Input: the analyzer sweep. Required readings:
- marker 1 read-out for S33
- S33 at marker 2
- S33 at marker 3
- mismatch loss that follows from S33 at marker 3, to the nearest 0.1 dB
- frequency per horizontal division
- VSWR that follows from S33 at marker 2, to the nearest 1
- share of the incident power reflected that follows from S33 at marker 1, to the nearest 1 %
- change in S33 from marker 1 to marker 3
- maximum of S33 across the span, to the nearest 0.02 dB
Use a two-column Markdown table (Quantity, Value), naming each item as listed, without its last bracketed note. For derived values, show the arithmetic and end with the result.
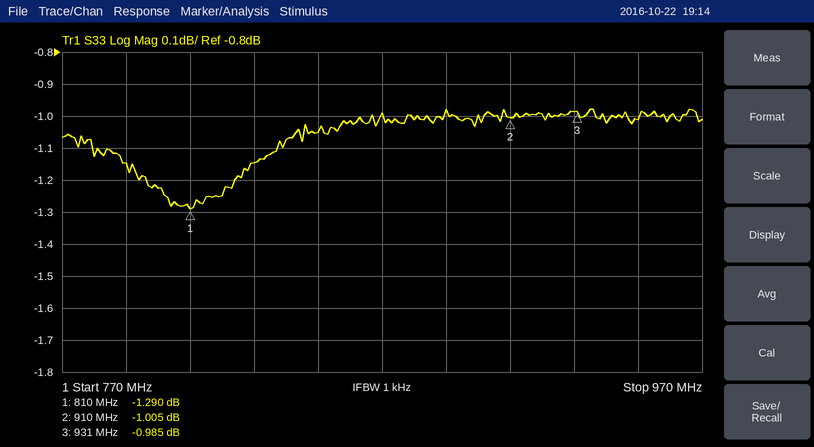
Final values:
| Quantity | Value |
|---|---|
| marker 1 read-out for S33 | -1.290 dB |
| S33 at marker 2 | -1.005 dB |
| S33 at marker 3 | -0.985 dB |
| mismatch loss that follows from S33 at marker 3, to the nearest 0.1 dB | −10 log10(1 − 10^(-0.985/10)) ≈ 6.9 dB |
| frequency per horizontal division | 20 MHz |
| VSWR that follows from S33 at marker 2, to the nearest 1 | (1 + 0.8907)/(1 − 0.8907) ≈ 17 |
| share of the incident power reflected that follows from S33 at marker 1, to the nearest 1 % | 10^(-1.29/10) ≈ 74 % |
| change in S33 from marker 1 to marker 3 | -0.985 − (-1.29) = 0.305 dB |
| maximum of S33 across the span, to the nearest 0.02 dB | -0.98 dB |
